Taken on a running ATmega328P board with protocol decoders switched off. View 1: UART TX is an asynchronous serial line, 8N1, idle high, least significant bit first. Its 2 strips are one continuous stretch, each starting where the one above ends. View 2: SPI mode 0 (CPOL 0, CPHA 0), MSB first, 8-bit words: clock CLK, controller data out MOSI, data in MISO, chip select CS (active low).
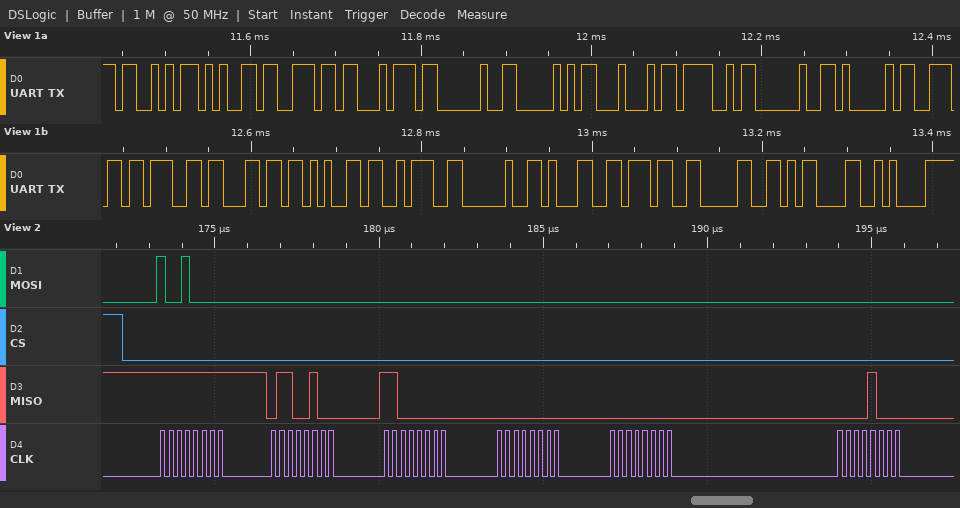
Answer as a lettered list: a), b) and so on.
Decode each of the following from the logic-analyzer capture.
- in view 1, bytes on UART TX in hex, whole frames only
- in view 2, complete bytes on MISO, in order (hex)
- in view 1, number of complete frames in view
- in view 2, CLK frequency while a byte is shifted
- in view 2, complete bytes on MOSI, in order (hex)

a) 53 65 6E 74 20 50 44 4F 20 41 6E 67 6C 65 3A 20 31 37 30 0D 0A
b) FF 64 C0 00 00 08
c) 21
d) 4 MHz
e) 90 00 00 00 00 00
